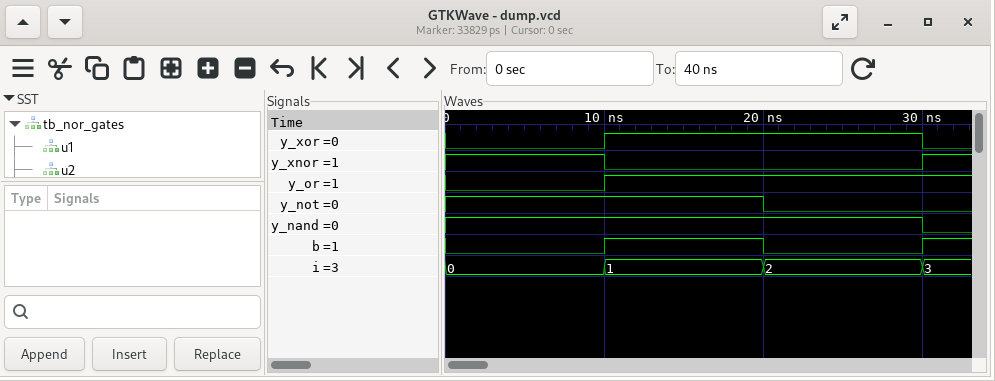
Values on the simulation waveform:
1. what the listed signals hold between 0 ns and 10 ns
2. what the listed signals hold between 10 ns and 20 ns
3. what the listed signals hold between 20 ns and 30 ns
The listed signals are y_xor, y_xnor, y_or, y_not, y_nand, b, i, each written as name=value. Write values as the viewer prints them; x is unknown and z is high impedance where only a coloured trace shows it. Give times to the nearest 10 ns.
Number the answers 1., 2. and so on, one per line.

1. y_xor=0, y_xnor=1, y_or=0, y_not=1, y_nand=1, b=0, i=0
2. y_xor=1, y_xnor=0, y_or=1, y_not=1, y_nand=1, b=1, i=1
3. y_xor=1, y_xnor=0, y_or=1, y_not=0, y_nand=1, b=0, i=2
